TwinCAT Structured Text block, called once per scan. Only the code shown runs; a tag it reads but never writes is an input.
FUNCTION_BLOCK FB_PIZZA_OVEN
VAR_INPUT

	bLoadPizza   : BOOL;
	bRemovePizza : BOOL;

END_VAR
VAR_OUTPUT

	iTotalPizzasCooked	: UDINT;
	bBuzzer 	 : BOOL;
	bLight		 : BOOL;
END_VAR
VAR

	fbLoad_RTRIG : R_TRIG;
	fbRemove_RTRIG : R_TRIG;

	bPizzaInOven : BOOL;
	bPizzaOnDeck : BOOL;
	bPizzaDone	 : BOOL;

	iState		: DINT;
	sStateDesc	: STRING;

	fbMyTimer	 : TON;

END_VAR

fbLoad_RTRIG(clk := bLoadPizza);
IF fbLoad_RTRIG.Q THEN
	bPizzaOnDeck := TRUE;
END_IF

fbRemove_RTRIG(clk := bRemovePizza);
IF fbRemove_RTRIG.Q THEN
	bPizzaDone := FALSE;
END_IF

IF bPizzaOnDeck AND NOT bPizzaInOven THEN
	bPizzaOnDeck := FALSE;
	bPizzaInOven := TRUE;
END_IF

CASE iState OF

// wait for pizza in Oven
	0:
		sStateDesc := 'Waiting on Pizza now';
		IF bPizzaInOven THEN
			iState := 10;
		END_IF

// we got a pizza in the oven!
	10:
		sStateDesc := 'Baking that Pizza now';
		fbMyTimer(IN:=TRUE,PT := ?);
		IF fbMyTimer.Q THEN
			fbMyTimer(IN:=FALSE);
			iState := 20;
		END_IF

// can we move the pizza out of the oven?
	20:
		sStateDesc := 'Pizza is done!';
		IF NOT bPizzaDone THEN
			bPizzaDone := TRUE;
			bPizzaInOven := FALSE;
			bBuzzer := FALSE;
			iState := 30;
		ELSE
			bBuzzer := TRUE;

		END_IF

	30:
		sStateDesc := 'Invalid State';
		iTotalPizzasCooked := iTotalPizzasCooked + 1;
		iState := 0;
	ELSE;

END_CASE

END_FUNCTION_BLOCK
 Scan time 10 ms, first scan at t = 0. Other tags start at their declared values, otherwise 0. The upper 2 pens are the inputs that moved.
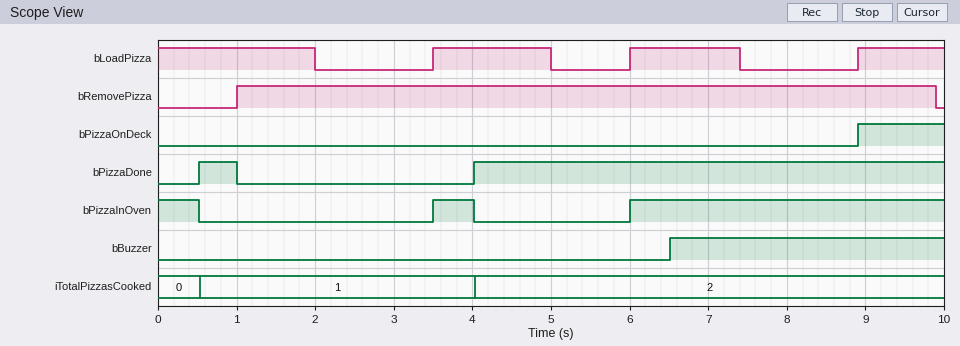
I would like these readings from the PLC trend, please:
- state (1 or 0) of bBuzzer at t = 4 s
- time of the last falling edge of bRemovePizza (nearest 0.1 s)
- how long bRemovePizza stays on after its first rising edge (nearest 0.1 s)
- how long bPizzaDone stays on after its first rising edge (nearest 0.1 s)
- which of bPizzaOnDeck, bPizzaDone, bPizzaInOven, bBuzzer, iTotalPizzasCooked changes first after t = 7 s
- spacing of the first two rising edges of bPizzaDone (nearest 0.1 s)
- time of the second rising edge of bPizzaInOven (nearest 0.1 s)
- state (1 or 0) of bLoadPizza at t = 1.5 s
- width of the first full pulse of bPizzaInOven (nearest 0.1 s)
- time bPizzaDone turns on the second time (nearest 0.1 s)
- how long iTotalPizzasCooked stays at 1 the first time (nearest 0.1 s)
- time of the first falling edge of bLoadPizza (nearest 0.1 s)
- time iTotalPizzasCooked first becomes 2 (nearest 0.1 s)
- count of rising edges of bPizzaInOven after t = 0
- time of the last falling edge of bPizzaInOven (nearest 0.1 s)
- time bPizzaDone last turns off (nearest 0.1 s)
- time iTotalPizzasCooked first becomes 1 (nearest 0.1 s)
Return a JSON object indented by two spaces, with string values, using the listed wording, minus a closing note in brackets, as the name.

{
  "state (1 or 0) of bBuzzer at t = 4 s": "0",
  "time of the last falling edge of bRemovePizza": "9.9 s",
  "how long bRemovePizza stays on after its first rising edge": "8.9 s",
  "how long bPizzaDone stays on after its first rising edge": "0.5 s",
  "which of bPizzaOnDeck, bPizzaDone, bPizzaInOven, bBuzzer, iTotalPizzasCooked changes first after t = 7 s": "bPizzaOnDeck",
  "spacing of the first two rising edges of bPizzaDone": "3.5 s",
  "time of the second rising edge of bPizzaInOven": "6.0 s",
  "state (1 or 0) of bLoadPizza at t = 1.5 s": "1",
  "width of the first full pulse of bPizzaInOven": "0.5 s",
  "time bPizzaDone turns on the second time": "4.0 s",
  "how long iTotalPizzasCooked stays at 1 the first time": "3.5 s",
  "time of the first falling edge of bLoadPizza": "2.0 s",
  "time iTotalPizzasCooked first becomes 2": "4.0 s",
  "count of rising edges of bPizzaInOven after t = 0": "2",
  "time of the last falling edge of bPizzaInOven": "4.0 s",
  "time bPizzaDone last turns off": "1.0 s",
  "time iTotalPizzasCooked first becomes 1": "0.5 s"
}
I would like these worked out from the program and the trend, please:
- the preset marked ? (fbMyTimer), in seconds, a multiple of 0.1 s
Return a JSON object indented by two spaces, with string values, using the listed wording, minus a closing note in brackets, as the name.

{
  "the preset marked ? (fbMyTimer), in seconds, a multiple of 0.1 s": "0.5 s"
}
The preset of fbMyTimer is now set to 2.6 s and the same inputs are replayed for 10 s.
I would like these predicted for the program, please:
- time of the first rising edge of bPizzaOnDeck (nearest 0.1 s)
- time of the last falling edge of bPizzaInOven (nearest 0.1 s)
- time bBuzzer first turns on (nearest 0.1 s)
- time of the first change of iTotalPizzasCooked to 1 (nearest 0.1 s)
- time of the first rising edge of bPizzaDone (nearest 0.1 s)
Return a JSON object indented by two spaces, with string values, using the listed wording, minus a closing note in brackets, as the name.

{
  "time of the first rising edge of bPizzaOnDeck": "6.0 s",
  "time of the last falling edge of bPizzaInOven": "2.6 s",
  "time bBuzzer first turns on": "6.1 s",
  "time of the first change of iTotalPizzasCooked to 1": "2.6 s",
  "time of the first rising edge of bPizzaDone": "2.6 s"
}
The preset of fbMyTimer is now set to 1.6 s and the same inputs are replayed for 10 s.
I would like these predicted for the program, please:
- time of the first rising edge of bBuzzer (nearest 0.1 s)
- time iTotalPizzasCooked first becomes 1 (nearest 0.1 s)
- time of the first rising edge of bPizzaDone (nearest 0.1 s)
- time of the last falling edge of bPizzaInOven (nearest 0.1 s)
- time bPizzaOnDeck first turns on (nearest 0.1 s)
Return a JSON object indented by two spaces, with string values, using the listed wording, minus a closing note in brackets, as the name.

{
  "time of the first rising edge of bBuzzer": "5.1 s",
  "time iTotalPizzasCooked first becomes 1": "1.6 s",
  "time of the first rising edge of bPizzaDone": "1.6 s",
  "time of the last falling edge of bPizzaInOven": "1.6 s",
  "time bPizzaOnDeck first turns on": "6.0 s"
}
